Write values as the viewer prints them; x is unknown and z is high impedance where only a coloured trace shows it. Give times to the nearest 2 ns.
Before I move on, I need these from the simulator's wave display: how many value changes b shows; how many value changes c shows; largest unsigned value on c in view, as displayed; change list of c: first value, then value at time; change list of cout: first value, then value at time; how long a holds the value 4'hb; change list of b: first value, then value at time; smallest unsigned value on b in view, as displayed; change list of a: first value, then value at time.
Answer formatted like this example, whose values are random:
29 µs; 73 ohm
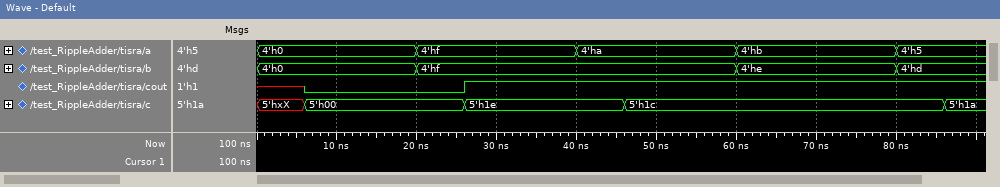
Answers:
3; 4; 5'h1e; 5'hxX, 5'h00 at 6 ns, 5'h1e at 26 ns, 5'h1c at 46 ns, 5'h1a at 86 ns; x, 0 at 6 ns, 1 at 26 ns; 20 ns; 4'h0, 4'hf at 20 ns, 4'he at 60 ns, 4'hd at 80 ns; 4'h0; 4'h0, 4'hf at 20 ns, 4'ha at 40 ns, 4'hb at 60 ns, 4'h5 at 80 ns
